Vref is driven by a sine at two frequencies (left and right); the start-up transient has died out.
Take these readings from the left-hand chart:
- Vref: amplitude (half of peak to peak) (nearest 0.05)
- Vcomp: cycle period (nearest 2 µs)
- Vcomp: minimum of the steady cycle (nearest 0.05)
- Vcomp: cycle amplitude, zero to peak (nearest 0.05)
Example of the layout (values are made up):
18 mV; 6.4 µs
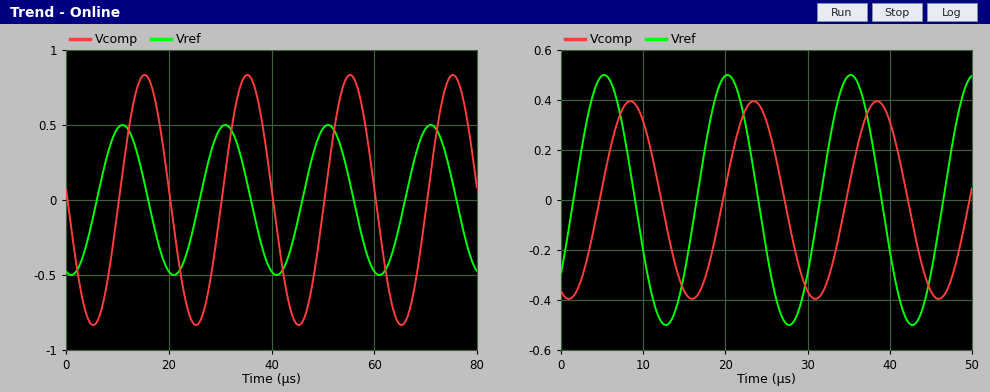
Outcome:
0.50; 20 µs; -0.85; 0.85
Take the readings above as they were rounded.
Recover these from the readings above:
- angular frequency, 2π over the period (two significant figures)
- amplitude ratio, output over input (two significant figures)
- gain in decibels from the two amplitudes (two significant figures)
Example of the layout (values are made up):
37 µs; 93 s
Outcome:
0.31 rad/µs; 1.7; 4.6 dB
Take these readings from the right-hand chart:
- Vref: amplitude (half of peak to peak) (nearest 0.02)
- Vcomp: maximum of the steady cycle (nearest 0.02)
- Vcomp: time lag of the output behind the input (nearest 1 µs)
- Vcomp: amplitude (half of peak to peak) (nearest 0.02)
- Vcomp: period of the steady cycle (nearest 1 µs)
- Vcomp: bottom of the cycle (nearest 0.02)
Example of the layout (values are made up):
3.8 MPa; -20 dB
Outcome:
0.50; 0.40; 3 µs; 0.40; 15 µs; -0.40
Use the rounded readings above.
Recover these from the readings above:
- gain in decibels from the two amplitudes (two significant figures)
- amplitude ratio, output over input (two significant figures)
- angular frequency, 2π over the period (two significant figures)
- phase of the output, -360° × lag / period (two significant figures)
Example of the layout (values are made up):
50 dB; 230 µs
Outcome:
-1.9 dB; 0.80; 0.42 rad/µs; -72°
